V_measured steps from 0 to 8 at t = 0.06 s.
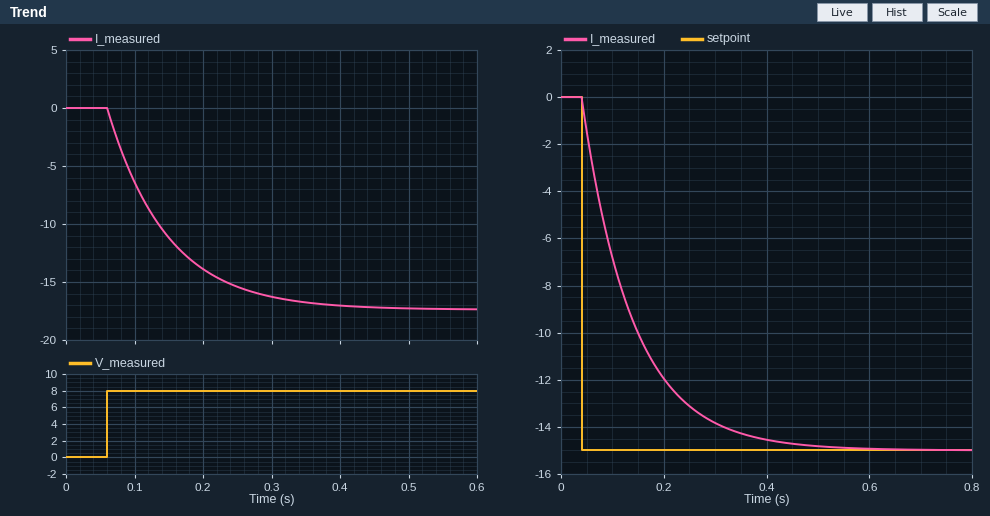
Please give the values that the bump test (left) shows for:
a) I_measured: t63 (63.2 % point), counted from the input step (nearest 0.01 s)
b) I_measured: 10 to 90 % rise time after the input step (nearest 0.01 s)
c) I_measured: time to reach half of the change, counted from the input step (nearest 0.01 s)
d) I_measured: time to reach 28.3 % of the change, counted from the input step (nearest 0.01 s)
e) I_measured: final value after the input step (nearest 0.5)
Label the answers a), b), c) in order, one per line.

a) 0.09 s
b) 0.19 s
c) 0.06 s
d) 0.03 s
e) -17.5
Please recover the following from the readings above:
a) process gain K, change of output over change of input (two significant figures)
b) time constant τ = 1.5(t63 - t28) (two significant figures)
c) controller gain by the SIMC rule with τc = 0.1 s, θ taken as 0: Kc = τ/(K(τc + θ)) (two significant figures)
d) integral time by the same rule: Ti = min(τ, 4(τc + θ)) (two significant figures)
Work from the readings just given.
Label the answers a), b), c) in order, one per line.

a) -2.2
b) 0.090 s
c) -0.41
d) 0.090 s
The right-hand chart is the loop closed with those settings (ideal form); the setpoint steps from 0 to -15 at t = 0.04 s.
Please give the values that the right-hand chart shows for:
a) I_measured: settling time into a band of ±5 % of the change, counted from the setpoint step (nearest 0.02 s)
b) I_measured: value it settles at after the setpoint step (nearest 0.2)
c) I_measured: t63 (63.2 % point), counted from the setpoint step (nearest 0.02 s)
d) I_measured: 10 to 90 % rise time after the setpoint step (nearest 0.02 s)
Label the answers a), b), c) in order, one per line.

a) 0.30 s
b) -15.0
c) 0.10 s
d) 0.22 s
